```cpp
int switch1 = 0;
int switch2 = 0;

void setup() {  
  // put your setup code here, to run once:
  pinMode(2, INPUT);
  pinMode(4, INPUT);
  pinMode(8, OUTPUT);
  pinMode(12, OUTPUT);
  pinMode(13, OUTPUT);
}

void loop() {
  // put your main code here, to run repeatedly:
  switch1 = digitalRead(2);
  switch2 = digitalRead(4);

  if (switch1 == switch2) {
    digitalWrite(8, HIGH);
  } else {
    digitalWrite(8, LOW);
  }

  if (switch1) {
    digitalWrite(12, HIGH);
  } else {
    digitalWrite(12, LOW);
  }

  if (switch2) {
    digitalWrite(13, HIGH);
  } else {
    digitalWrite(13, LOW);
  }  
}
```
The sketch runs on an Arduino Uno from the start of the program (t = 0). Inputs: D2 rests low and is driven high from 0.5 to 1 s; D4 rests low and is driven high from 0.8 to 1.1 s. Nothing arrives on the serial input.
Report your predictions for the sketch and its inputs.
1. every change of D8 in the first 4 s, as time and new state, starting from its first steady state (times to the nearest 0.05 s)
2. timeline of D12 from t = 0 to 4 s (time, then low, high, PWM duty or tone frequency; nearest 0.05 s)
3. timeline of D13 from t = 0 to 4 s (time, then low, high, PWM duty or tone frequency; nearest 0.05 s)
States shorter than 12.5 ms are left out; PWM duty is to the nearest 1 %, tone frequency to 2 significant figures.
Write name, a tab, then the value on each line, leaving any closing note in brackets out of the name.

every change of D8 in the first 4 s, as time and new state, starting from its first steady state	0 s high; 0.5 s low; 0.8 s high; 1 s low; 1.1 s high
timeline of D12 from t = 0 to 4 s	0 s low; 0.5 s high; 1 s low
timeline of D13 from t = 0 to 4 s	0 s low; 0.8 s high; 1.1 s low
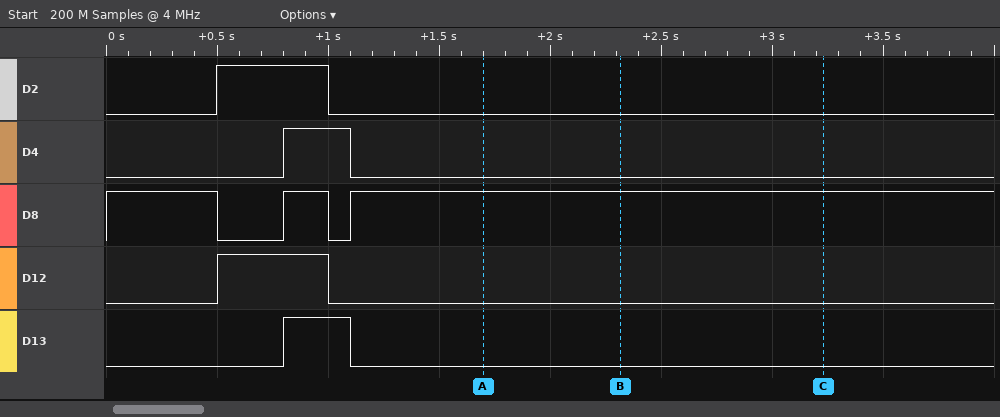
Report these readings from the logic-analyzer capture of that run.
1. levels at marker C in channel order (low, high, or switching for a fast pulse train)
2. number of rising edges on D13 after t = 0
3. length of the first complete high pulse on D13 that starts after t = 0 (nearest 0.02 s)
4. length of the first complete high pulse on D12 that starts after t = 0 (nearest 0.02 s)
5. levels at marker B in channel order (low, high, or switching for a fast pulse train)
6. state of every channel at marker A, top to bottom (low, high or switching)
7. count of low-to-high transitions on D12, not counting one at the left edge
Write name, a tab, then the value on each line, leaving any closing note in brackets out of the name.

levels at marker C in channel order	D2 low, D4 low, D8 high, D12 low, D13 low
number of rising edges on D13 after t = 0	1
length of the first complete high pulse on D13 that starts after t = 0	0.30 s
length of the first complete high pulse on D12 that starts after t = 0	0.50 s
levels at marker B in channel order	D2 low, D4 low, D8 high, D12 low, D13 low
state of every channel at marker A, top to bottom	D2 low, D4 low, D8 high, D12 low, D13 low
count of low-to-high transitions on D12, not counting one at the left edge	1
